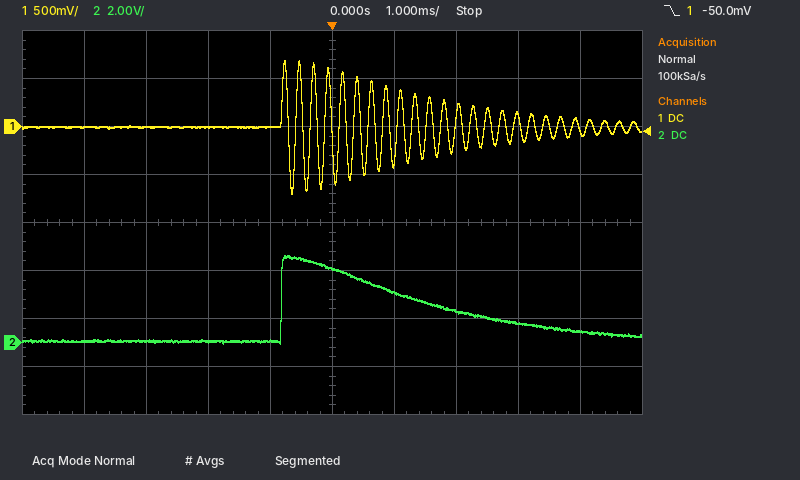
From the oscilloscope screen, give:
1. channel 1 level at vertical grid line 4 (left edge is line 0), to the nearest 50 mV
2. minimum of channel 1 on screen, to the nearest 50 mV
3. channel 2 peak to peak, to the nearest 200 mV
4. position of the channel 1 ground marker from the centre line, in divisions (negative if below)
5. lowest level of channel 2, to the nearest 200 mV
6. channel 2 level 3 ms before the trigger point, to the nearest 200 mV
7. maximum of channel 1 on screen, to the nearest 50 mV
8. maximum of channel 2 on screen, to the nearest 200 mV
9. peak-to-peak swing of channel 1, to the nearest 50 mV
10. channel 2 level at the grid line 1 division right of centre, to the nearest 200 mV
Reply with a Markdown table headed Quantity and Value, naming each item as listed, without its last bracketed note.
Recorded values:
| Quantity | Value |
|---|---|
| channel 1 level at vertical grid line 4 (left edge is line 0), to the nearest 50 mV | 0 mV |
| minimum of channel 1 on screen, to the nearest 50 mV | -700 mV |
| channel 2 peak to peak, to the nearest 200 mV | 3.6 V |
| position of the channel 1 ground marker from the centre line, in divisions | +2.0 div |
| lowest level of channel 2, to the nearest 200 mV | 0.0 V |
| channel 2 level 3 ms before the trigger point, to the nearest 200 mV | 0.0 V |
| maximum of channel 1 on screen, to the nearest 50 mV | 700 mV |
| maximum of channel 2 on screen, to the nearest 200 mV | 3.6 V |
| peak-to-peak swing of channel 1, to the nearest 50 mV | 1.40 V |
| channel 2 level at the grid line 1 division right of centre, to the nearest 200 mV | 2.0 V |
